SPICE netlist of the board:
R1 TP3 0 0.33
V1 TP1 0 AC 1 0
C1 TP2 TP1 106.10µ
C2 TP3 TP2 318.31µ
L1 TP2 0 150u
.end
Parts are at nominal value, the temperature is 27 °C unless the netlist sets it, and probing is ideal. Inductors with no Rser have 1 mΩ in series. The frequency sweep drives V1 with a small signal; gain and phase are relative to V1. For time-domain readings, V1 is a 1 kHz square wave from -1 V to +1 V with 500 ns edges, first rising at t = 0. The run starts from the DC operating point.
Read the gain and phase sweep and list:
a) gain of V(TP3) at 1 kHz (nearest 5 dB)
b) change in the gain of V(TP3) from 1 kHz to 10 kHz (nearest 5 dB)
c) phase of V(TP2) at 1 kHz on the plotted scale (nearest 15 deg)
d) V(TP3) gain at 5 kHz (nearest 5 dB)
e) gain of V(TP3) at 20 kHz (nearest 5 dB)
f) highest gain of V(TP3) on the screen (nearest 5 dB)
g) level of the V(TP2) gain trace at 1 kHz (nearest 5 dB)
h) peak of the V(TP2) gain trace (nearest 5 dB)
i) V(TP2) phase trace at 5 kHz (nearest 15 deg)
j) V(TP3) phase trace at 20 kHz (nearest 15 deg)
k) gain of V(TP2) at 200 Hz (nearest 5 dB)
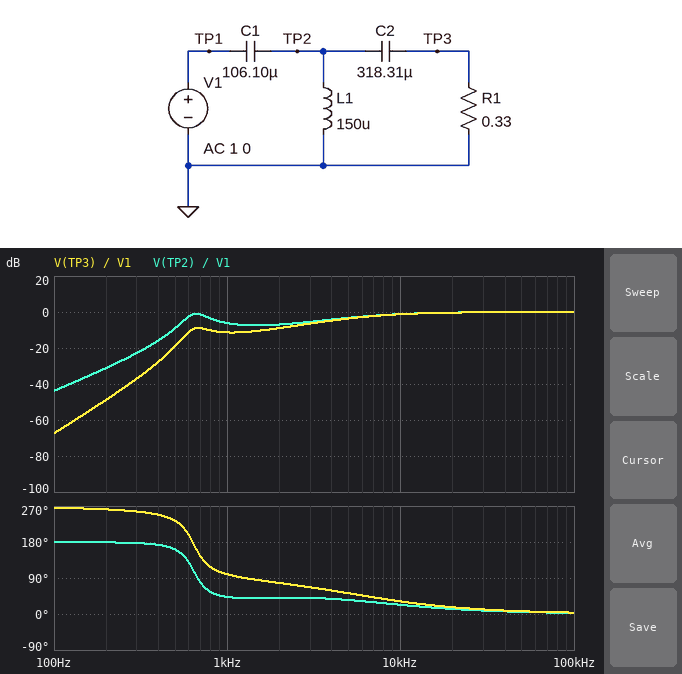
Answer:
-10 dB
10 dB
45 deg
-5 dB
0 dB
0 dB
-5 dB
0 dB
30 deg
15 deg
-30 dB
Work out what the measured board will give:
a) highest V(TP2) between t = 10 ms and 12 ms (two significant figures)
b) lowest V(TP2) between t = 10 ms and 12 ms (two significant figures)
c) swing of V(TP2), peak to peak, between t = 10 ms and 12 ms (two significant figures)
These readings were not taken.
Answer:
2.0 V
-2.0 V
4.1 V
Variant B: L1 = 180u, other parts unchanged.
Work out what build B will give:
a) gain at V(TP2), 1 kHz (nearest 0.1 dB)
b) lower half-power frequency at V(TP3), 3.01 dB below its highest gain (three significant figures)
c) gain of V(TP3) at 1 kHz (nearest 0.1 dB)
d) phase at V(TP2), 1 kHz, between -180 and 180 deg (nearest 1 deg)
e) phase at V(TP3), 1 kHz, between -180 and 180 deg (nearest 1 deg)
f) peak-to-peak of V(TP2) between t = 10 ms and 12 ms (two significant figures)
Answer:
-7.0 dB
5.78 kHz
-12.2 dB
38 deg
95 deg
3.9 V
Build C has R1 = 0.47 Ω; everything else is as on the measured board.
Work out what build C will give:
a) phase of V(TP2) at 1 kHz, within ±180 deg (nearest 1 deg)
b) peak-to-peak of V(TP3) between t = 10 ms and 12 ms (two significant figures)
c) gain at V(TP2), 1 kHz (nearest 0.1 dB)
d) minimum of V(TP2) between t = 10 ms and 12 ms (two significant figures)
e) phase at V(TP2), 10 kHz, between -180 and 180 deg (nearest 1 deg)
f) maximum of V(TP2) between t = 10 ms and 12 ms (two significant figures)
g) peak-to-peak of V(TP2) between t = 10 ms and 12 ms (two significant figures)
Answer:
56 deg
4.4 V
-5.1 dB
-2.2 V
17 deg
2.2 V
4.3 V
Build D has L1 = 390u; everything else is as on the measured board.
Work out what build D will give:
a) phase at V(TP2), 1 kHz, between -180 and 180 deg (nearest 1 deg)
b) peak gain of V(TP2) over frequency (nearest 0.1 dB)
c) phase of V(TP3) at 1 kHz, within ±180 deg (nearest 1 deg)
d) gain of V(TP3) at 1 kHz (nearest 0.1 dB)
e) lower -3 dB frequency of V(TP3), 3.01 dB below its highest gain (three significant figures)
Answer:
29 deg
2.6 dB
86 deg
-14.2 dB
5.93 kHz
